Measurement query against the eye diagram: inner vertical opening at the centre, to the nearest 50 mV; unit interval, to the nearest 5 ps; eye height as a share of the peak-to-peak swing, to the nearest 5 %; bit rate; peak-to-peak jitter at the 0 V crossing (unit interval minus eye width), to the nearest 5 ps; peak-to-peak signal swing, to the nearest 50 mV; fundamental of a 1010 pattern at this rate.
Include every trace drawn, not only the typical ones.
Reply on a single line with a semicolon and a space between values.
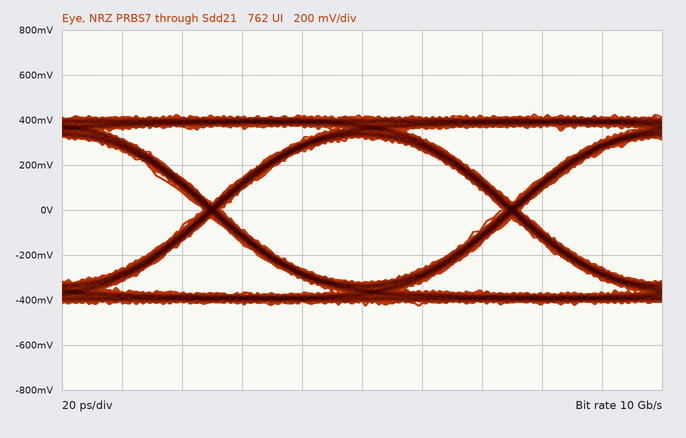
650 mV; 100 ps; 75 %; 10 Gb/s; 5 ps; 850 mV; 5 GHz
